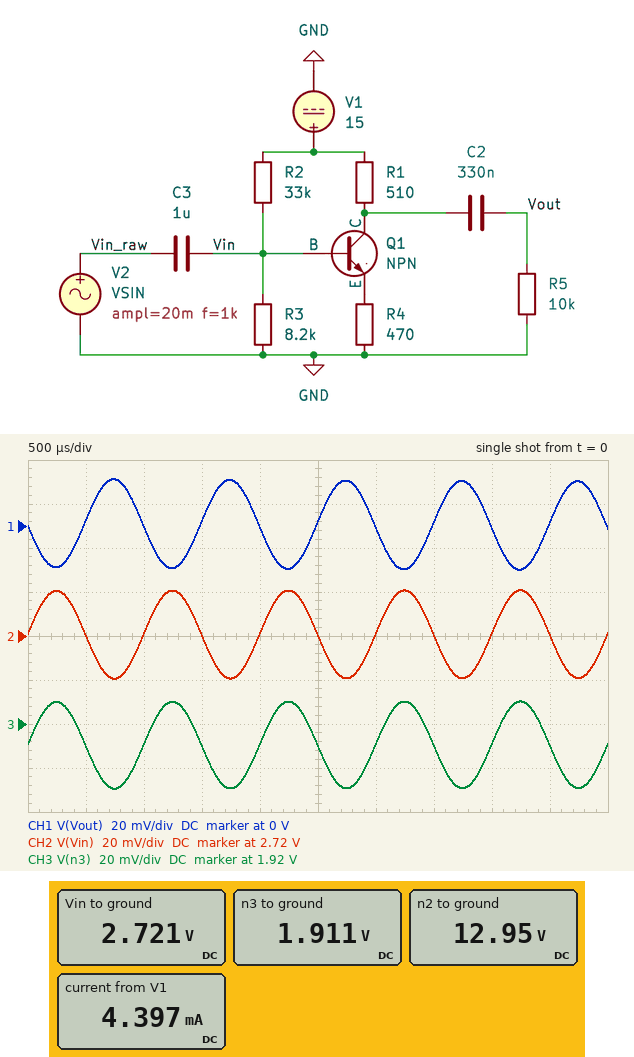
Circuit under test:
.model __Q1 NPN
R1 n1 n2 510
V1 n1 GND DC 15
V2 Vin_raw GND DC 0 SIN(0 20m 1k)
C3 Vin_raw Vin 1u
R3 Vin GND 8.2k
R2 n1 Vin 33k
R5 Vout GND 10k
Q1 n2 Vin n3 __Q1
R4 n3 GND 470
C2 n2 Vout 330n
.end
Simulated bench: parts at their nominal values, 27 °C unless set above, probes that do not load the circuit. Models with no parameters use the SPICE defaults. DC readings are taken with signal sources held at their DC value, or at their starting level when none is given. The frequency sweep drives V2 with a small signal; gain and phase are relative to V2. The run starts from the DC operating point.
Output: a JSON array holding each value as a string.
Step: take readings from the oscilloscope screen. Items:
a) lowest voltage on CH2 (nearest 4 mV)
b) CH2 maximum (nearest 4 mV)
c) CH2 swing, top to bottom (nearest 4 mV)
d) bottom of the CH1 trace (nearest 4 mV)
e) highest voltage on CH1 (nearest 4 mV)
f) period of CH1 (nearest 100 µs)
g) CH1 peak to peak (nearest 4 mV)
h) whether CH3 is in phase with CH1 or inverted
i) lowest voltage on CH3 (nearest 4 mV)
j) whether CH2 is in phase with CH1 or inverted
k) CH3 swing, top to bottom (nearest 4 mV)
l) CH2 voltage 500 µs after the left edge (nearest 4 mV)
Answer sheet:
["2.700 V", "2.740 V", "40 mV", "-20 mV", "20 mV", "1.0 ms", "40 mV", "inverted", "1.892 V", "inverted", "40 mV", "2.720 V"]
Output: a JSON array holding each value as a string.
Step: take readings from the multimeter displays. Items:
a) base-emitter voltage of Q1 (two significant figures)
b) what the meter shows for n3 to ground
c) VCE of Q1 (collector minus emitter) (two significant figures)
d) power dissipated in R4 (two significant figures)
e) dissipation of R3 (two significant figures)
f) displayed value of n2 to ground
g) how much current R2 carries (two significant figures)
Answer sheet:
["810 mV", "1.911 V", "11 V", "7.8 mW", "900 µW", "12.95 V", "370 µA"]
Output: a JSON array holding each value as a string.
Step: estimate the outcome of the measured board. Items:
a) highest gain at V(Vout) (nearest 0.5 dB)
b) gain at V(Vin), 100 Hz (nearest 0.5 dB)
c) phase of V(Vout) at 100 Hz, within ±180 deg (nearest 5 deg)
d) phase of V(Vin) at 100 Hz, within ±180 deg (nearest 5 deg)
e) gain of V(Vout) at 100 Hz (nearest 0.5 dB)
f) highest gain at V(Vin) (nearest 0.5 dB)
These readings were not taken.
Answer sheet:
["0 dB", "-0.5 dB", "-140 deg", "15 deg", "-1.0 dB", "0 dB"]
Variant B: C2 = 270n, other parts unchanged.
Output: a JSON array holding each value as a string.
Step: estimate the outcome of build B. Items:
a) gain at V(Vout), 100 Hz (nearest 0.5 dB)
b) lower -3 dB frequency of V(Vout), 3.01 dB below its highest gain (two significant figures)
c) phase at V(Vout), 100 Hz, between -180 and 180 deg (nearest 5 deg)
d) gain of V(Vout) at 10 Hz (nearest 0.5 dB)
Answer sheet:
["-1.5 dB", "67 Hz", "-135 deg", "-24.5 dB"]
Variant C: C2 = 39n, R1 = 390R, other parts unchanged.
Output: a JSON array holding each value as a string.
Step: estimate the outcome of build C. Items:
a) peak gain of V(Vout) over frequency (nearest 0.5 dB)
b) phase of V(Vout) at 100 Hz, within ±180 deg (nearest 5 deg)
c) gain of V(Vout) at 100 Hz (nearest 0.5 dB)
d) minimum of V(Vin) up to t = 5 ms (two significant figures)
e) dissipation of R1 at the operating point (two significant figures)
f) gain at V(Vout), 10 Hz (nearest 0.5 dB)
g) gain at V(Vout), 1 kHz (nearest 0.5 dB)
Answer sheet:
["-2.0 dB", "-90 deg", "-14.5 dB", "2.7 V", "6.3 mW", "-43.5 dB", "-3.0 dB"]
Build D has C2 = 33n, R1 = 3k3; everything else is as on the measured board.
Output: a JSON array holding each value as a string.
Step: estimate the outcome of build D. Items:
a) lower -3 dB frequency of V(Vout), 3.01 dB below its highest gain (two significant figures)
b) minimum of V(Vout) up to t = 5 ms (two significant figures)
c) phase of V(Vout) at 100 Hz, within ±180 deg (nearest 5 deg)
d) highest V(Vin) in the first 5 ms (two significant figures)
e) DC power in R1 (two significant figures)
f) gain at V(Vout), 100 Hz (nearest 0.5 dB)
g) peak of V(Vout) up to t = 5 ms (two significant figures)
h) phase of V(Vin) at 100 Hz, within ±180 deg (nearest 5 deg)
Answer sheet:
["470 Hz", "-61 mV", "-40 deg", "2.7 V", "51 mW", "-11.5 dB", "84 mV", "65 deg"]
